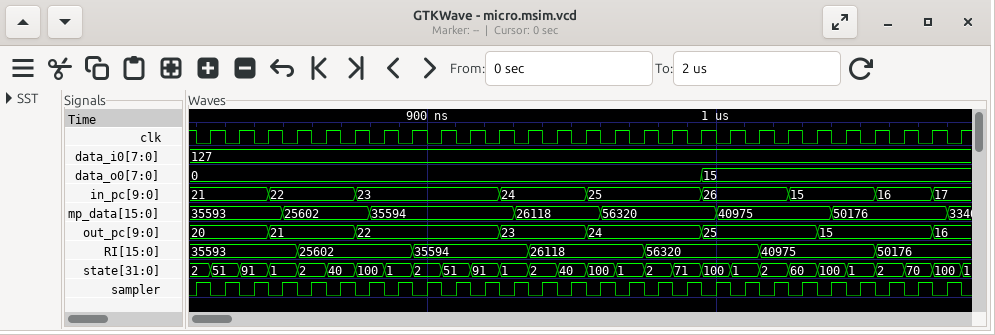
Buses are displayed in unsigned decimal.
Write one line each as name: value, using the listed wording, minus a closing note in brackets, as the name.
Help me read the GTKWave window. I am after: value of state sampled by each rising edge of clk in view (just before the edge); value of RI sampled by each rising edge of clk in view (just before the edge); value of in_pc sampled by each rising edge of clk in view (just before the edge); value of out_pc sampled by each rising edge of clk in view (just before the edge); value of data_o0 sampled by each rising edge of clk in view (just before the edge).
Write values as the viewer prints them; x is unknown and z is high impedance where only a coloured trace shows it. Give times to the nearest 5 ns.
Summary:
value of state sampled by each rising edge of clk in view: 2, 51, 91, 1, 2, 40, 100, 1, 2, 51, 91, 1, 2, 40, 100, 1, 2, 71, 100, 1, 2, 60, 100, 1, 2, 70, 100
value of RI sampled by each rising edge of clk in view: 35593, 35593, 35593, 35593, 25602, 25602, 25602, 25602, 35594, 35594, 35594, 35594, 26118, 26118, 26118, 26118, 56320, 56320, 56320, 56320, 40975, 40975, 40975, 40975, 50176, 50176, 50176
value of in_pc sampled by each rising edge of clk in view: 21, 21, 21, 22, 22, 22, 23, 23, 23, 23, 23, 24, 24, 24, 25, 25, 25, 25, 26, 26, 26, 15, 15, 15, 16, 16, 17
value of out_pc sampled by each rising edge of clk in view: 20, 20, 20, 21, 21, 21, 22, 22, 22, 22, 22, 23, 23, 23, 24, 24, 24, 24, 25, 25, 25, 25, 15, 15, 15, 15, 16
value of data_o0 sampled by each rising edge of clk in view: 0, 0, 0, 0, 0, 0, 0, 0, 0, 0, 0, 0, 0, 0, 0, 0, 0, 0, 15, 15, 15, 15, 15, 15, 15, 15, 15
